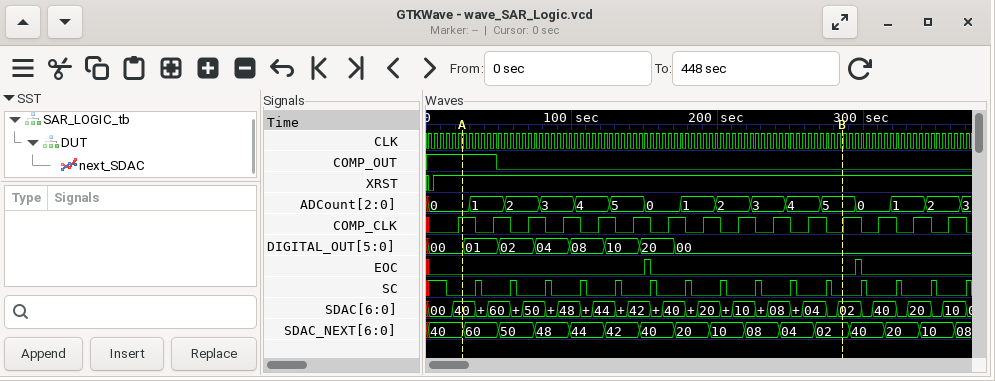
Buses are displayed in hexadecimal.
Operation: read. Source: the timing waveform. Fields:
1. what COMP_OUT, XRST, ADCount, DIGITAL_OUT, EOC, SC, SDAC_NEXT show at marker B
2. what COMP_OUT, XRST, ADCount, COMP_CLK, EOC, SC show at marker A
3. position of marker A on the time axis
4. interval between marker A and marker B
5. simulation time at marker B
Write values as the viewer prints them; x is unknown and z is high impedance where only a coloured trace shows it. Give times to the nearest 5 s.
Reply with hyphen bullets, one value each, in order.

- COMP_OUT=0, XRST=1, ADCount=5, DIGITAL_OUT=00, EOC=0, SC=0, SDAC_NEXT=02
- COMP_OUT=1, XRST=1, ADCount=0, COMP_CLK=1, EOC=0, SC=0
- 25 s
- 260 s
- 285 s
